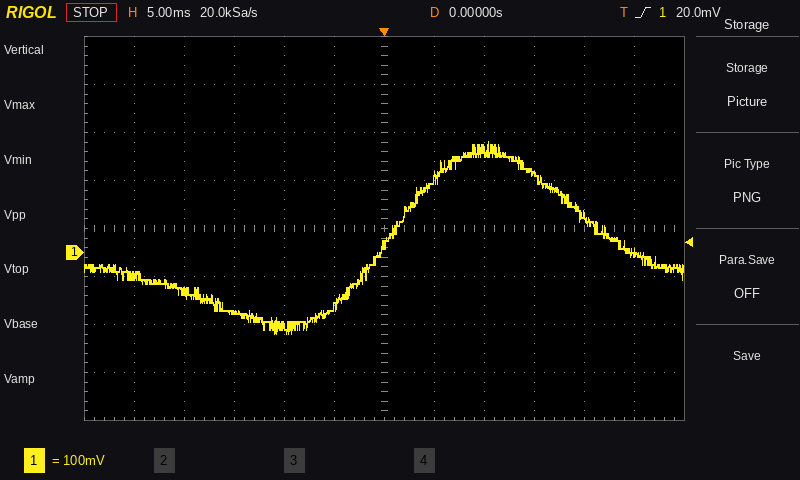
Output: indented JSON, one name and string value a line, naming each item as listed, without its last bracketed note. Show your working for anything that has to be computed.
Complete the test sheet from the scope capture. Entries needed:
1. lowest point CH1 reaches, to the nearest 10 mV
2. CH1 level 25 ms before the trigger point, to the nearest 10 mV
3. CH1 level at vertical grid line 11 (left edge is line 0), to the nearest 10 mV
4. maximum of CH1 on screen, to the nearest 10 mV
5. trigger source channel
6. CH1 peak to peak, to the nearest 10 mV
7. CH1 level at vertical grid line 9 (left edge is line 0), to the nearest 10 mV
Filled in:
{
  "lowest point CH1 reaches, to the nearest 10 mV": "-170 mV",
  "CH1 level 25 ms before the trigger point, to the nearest 10 mV": "-50 mV",
  "CH1 level at vertical grid line 11 (left edge is line 0), to the nearest 10 mV": "0 mV",
  "maximum of CH1 on screen, to the nearest 10 mV": "230 mV",
  "trigger source channel": "CH1",
  "CH1 peak to peak, to the nearest 10 mV": "230 mV − (-170 mV) = 400 mV",
  "CH1 level at vertical grid line 9 (left edge is line 0), to the nearest 10 mV": "170 mV"
}
